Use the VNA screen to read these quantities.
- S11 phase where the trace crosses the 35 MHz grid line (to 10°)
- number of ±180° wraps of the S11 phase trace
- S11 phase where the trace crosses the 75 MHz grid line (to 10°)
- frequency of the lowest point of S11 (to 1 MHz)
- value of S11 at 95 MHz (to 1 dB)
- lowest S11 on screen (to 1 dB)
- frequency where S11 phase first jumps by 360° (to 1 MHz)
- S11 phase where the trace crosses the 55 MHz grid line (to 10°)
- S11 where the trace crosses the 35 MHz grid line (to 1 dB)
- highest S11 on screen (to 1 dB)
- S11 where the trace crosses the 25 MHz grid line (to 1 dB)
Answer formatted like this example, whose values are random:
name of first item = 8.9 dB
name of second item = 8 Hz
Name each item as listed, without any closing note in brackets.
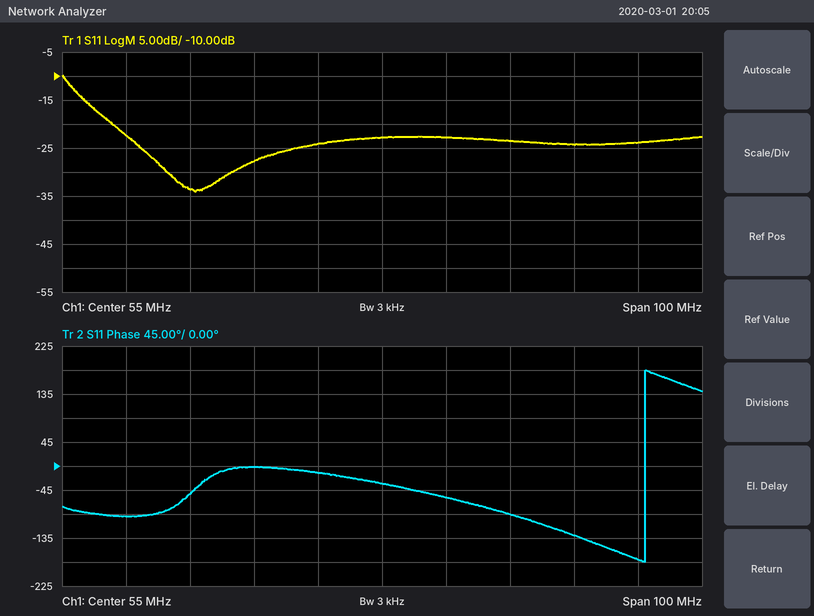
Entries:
S11 phase where the trace crosses the 35 MHz grid line = 0°
number of ±180° wraps of the S11 phase trace = 1
S11 phase where the trace crosses the 75 MHz grid line = -90°
frequency of the lowest point of S11 = 26 MHz
value of S11 at 95 MHz = -24 dB
lowest S11 on screen = -34 dB
frequency where S11 phase first jumps by 360° = 96 MHz
S11 phase where the trace crosses the 55 MHz grid line = -30°
S11 where the trace crosses the 35 MHz grid line = -28 dB
highest S11 on screen = -10 dB
S11 where the trace crosses the 25 MHz grid line = -34 dB
